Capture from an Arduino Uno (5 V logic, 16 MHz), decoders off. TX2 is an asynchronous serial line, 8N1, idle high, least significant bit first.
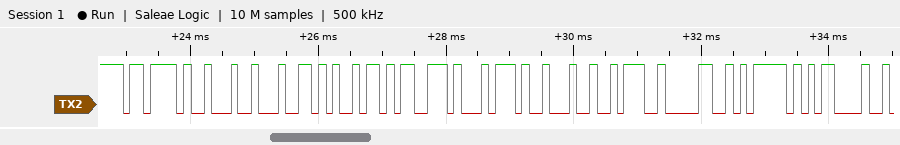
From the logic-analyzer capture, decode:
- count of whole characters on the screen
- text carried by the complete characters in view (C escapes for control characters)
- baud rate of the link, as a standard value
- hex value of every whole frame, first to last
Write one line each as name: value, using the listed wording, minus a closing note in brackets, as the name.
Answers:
count of whole characters on the screen: 11
text carried by the complete characters in view: "{\"dist\":0}\r"
baud rate of the link, as a standard value: 9600 baud
hex value of every whole frame, first to last: 0x7B 0x22 0x64 0x69 0x73 0x74 0x22 0x3A 0x30 0x7D 0x0D
